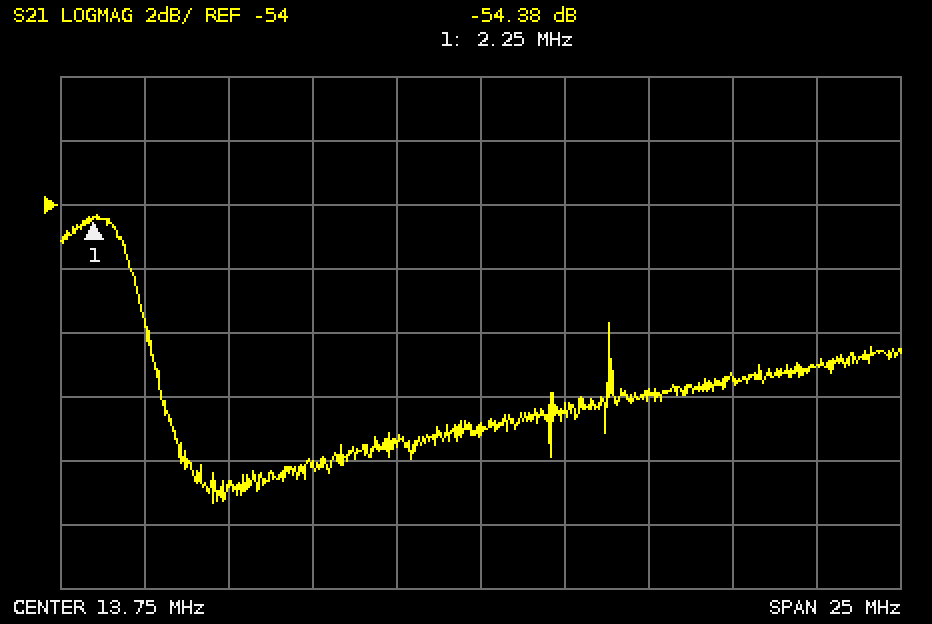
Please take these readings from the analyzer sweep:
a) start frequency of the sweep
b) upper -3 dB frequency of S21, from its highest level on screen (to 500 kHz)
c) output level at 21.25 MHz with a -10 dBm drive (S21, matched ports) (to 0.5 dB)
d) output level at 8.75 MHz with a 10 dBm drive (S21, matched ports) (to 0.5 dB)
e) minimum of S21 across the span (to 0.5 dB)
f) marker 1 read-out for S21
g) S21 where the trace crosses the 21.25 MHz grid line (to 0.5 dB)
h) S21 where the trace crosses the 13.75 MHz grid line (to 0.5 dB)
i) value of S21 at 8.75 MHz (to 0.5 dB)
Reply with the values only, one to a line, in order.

1.25 MHz
3.5 MHz
-69.5 dBm
-52.0 dBm
-63.5 dB
-54.38 dB
-59.5 dB
-61.0 dB
-62.0 dB
